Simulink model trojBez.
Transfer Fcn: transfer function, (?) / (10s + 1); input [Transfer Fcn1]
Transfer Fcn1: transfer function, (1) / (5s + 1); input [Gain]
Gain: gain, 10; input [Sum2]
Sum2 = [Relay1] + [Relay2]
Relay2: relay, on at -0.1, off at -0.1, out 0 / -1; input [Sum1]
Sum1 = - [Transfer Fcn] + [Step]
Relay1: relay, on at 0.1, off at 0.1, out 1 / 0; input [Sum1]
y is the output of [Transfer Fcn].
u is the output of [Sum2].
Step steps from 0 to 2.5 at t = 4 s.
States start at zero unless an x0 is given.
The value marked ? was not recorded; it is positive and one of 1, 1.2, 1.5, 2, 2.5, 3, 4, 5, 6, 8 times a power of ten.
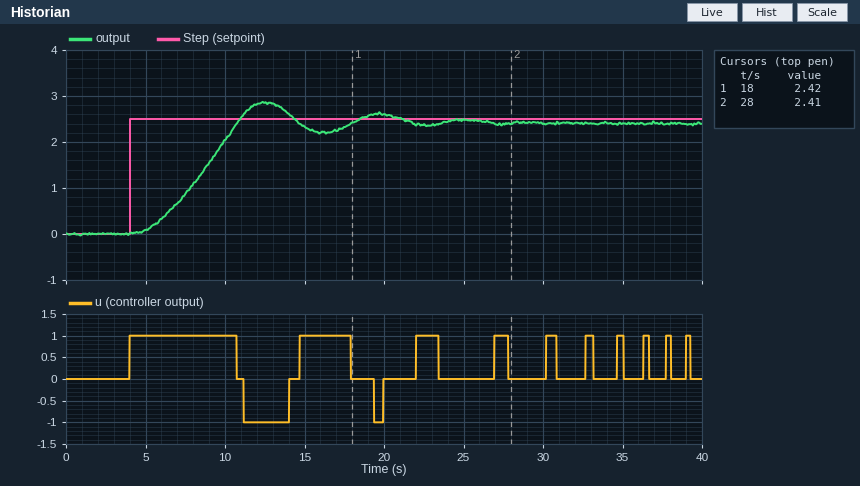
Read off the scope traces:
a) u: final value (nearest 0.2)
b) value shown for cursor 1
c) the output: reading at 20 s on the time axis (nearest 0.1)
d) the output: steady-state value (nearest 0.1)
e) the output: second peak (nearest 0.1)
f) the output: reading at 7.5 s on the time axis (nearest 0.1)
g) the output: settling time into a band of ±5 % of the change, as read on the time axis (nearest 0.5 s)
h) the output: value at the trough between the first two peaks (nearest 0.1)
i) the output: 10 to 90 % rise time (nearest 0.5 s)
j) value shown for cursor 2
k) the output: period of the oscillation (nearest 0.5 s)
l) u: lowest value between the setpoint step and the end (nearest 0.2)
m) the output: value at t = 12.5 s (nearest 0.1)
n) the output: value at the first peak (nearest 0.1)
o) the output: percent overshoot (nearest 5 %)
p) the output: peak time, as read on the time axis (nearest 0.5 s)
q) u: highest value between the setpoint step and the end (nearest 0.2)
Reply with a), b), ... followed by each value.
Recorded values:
a) 0.0
b) 2.42
c) 2.6
d) 2.4
e) 2.6
f) 0.9
g) 21.0 s
h) 2.2
i) 4.5 s
j) 2.41
k) 7.0 s
l) -1.0
m) 2.9
n) 2.9
o) 20 %
p) 12.5 s
q) 1.0
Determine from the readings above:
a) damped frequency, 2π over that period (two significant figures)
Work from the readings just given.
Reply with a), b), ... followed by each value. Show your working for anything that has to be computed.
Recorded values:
a) 2π / 7 = 0.90 rad/s
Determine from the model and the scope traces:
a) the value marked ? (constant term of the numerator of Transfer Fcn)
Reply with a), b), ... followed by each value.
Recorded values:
a) 1
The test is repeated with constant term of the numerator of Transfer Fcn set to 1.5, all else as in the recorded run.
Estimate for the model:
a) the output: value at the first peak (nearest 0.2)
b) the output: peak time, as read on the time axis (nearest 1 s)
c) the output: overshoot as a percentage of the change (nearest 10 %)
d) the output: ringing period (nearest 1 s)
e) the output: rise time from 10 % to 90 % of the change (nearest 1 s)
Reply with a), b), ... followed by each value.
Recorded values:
a) 3.0
b) 11 s
c) 30 %
d) 6 s
e) 3 s
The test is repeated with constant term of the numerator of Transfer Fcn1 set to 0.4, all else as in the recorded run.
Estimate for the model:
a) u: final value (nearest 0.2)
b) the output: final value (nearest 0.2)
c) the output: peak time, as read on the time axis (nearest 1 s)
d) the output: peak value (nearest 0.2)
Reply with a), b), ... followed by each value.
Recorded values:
a) 1.0
b) 2.4
c) 21 s
d) 2.6
